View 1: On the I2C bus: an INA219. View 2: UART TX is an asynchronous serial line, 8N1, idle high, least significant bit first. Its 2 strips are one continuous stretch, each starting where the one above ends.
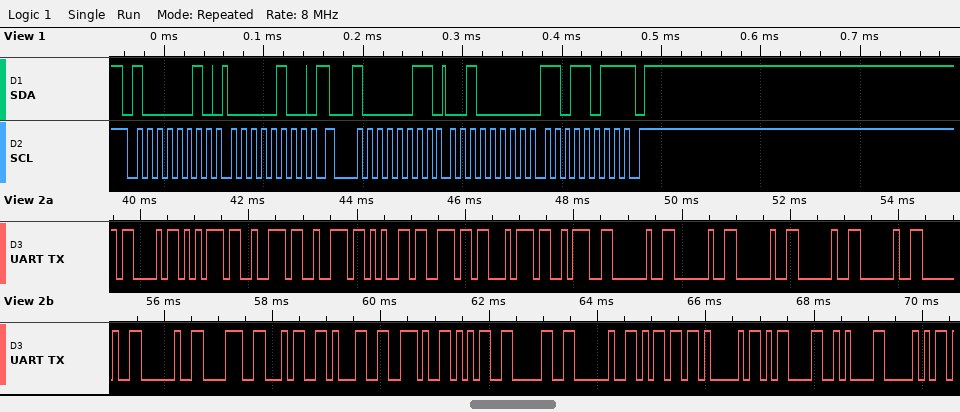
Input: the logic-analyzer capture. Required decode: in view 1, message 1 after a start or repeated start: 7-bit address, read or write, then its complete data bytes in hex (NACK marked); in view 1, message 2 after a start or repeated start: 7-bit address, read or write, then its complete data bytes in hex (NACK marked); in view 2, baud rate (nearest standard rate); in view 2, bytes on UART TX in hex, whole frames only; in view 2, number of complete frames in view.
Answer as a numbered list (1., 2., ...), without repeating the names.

1. 0x41 write: 04
2. 0x41 read: 20 DB NACK
3. 9600 baud
4. 0x43 0x75 0x72 0x72 0x65 0x6E 0x74 0x3A 0x20 0x20 0x20 0x20 0x20 0x20 0x20 0x38 0x34 0x31 0x2E 0x35 0x30 0x20 0x6D 0x41 0x0D 0x0A 0x50
5. 27
